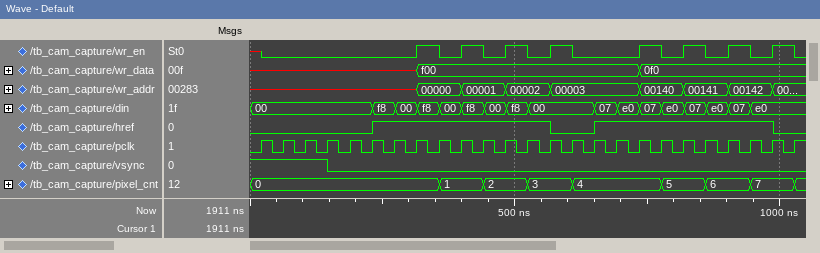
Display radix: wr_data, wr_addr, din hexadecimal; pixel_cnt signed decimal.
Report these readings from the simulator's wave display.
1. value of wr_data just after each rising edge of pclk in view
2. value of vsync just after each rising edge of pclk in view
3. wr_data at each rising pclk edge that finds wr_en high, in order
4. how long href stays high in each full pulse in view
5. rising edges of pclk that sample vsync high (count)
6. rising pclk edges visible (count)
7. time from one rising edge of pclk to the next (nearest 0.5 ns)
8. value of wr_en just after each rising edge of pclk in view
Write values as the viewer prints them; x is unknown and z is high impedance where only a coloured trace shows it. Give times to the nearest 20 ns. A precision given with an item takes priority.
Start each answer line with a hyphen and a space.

- x, x, x, x, x, x, x, f00, f00, f00, f00, f00, f00, f00, f00, f00, f00, 0f0, 0f0, 0f0, 0f0, 0f0, 0f0, 0f0, 0f0
- 1 1 1 0 0 0 0 0 0 0 0 0 0 0 0 0 0 0 0 0 0 0 0 0 0
- f00, f00, f00, f00, 0f0, 0f0, 0f0, 0f0
- 340 ns, 340 ns
- 4
- 25
- 42 ns
- 0 0 0 0 0 0 0 1 0 1 0 1 0 1 0 0 0 1 0 1 0 1 0 1 0
